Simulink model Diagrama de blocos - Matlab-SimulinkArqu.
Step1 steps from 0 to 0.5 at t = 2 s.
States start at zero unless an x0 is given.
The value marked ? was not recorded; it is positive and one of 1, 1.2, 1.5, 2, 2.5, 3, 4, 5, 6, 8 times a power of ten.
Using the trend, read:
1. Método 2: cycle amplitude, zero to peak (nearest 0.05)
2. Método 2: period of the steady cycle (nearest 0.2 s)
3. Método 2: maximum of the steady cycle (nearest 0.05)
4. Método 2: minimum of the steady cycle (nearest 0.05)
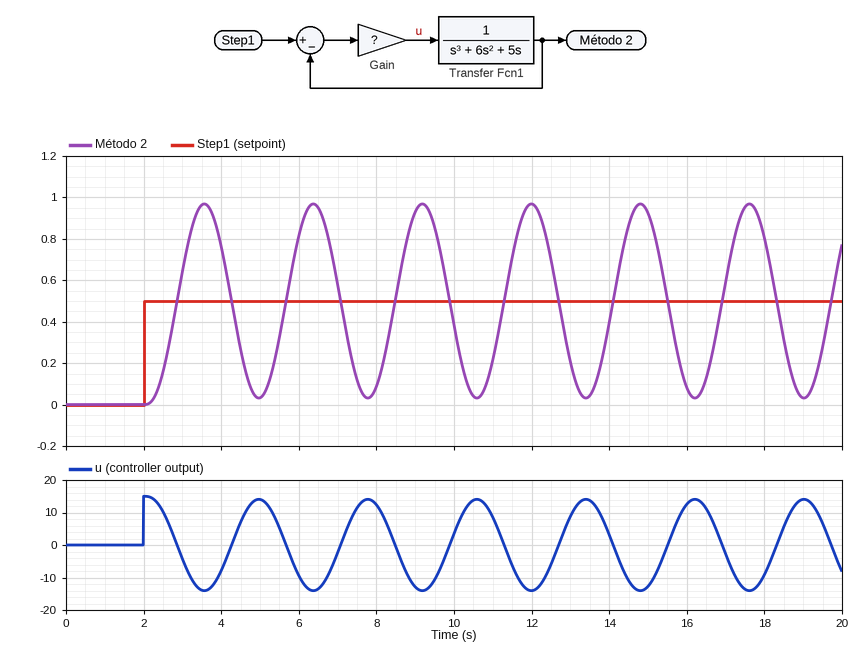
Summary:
0.45
2.8 s
0.95
0.05
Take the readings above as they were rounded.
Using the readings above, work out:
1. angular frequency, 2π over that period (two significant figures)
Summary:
2.2 rad/s
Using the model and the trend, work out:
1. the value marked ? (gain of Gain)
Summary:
30
